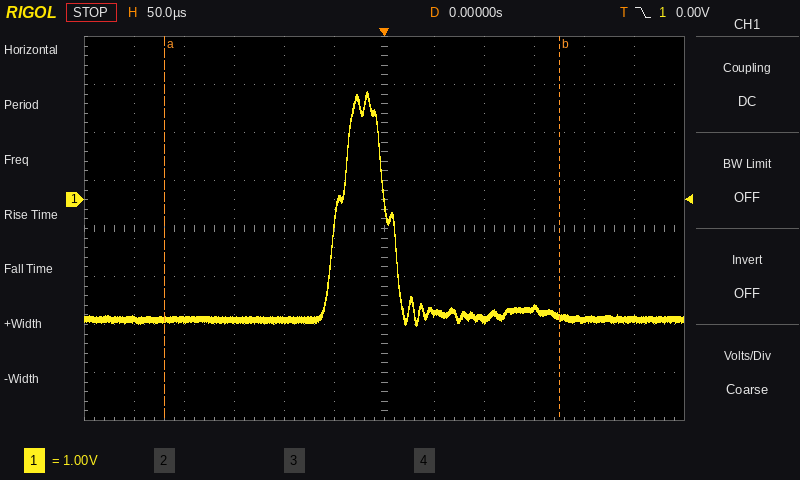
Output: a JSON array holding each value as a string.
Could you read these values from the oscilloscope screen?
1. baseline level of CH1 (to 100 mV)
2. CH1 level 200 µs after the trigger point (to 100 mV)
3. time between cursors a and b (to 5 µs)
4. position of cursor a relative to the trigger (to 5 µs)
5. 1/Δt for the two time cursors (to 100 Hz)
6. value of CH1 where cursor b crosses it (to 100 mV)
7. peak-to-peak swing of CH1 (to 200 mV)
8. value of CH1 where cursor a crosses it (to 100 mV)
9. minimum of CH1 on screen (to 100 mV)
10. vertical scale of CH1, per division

["-2.5 V", "-2.5 V", "395 µs", "-220 µs", "2.5 kHz", "-2.4 V", "4.8 V", "-2.5 V", "-2.6 V", "1 V"]
